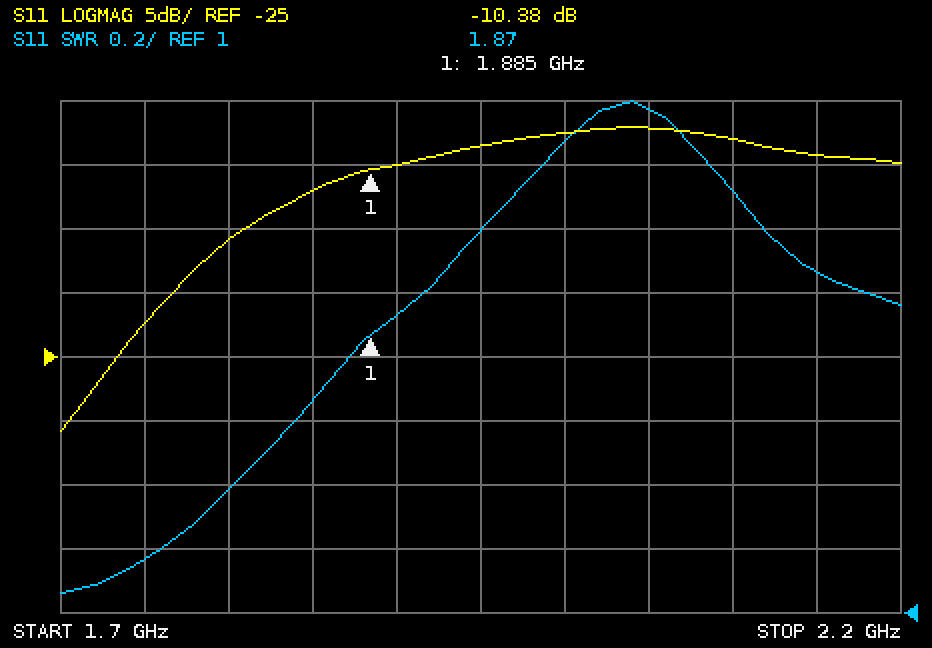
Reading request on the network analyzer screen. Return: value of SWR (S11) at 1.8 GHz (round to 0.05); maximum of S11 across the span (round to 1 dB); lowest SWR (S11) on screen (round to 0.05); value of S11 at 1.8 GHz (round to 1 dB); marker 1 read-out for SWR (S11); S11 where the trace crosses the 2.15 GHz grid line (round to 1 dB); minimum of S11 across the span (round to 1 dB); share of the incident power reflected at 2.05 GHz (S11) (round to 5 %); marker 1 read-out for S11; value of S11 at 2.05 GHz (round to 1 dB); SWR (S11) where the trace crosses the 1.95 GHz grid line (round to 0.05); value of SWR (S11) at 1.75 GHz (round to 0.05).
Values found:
1.40
-7 dB
1.05
-16 dB
1.87
-9 dB
-31 dB
20 %
-10.38 dB
-7 dB
2.20
1.15
